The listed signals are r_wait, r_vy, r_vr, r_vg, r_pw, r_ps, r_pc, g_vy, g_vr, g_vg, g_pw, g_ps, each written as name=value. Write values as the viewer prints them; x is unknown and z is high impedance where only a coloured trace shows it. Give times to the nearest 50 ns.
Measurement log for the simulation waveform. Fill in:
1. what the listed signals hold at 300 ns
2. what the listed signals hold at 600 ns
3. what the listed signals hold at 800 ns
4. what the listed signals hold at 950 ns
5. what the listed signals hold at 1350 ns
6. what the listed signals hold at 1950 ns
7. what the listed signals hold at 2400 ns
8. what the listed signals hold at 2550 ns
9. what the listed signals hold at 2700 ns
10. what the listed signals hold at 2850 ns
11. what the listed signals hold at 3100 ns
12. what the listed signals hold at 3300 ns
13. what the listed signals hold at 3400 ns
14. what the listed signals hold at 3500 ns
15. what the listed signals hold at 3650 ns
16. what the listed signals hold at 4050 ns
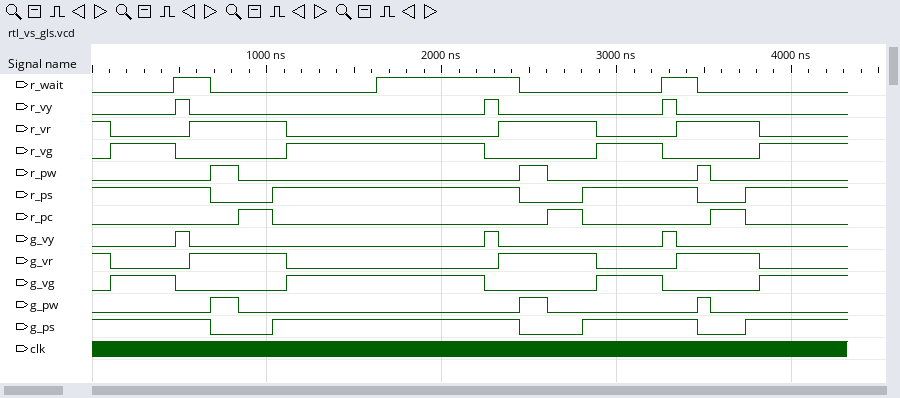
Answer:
r_wait=0, r_vy=0, r_vr=0, r_vg=1, r_pw=0, r_ps=1, r_pc=0, g_vy=0, g_vr=0, g_vg=1, g_pw=0, g_ps=1
r_wait=1, r_vy=0, r_vr=1, r_vg=0, r_pw=0, r_ps=1, r_pc=0, g_vy=0, g_vr=1, g_vg=0, g_pw=0, g_ps=1
r_wait=0, r_vy=0, r_vr=1, r_vg=0, r_pw=1, r_ps=0, r_pc=0, g_vy=0, g_vr=1, g_vg=0, g_pw=1, g_ps=0
r_wait=0, r_vy=0, r_vr=1, r_vg=0, r_pw=0, r_ps=0, r_pc=1, g_vy=0, g_vr=1, g_vg=0, g_pw=0, g_ps=0
r_wait=0, r_vy=0, r_vr=0, r_vg=1, r_pw=0, r_ps=1, r_pc=0, g_vy=0, g_vr=0, g_vg=1, g_pw=0, g_ps=1
r_wait=1, r_vy=0, r_vr=0, r_vg=1, r_pw=0, r_ps=1, r_pc=0, g_vy=0, g_vr=0, g_vg=1, g_pw=0, g_ps=1
r_wait=1, r_vy=0, r_vr=1, r_vg=0, r_pw=0, r_ps=1, r_pc=0, g_vy=0, g_vr=1, g_vg=0, g_pw=0, g_ps=1
r_wait=0, r_vy=0, r_vr=1, r_vg=0, r_pw=1, r_ps=0, r_pc=0, g_vy=0, g_vr=1, g_vg=0, g_pw=1, g_ps=0
r_wait=0, r_vy=0, r_vr=1, r_vg=0, r_pw=0, r_ps=0, r_pc=1, g_vy=0, g_vr=1, g_vg=0, g_pw=0, g_ps=0
r_wait=0, r_vy=0, r_vr=1, r_vg=0, r_pw=0, r_ps=1, r_pc=0, g_vy=0, g_vr=1, g_vg=0, g_pw=0, g_ps=1
r_wait=0, r_vy=0, r_vr=0, r_vg=1, r_pw=0, r_ps=1, r_pc=0, g_vy=0, g_vr=0, g_vg=1, g_pw=0, g_ps=1
r_wait=1, r_vy=1, r_vr=0, r_vg=0, r_pw=0, r_ps=1, r_pc=0, g_vy=1, g_vr=0, g_vg=0, g_pw=0, g_ps=1
r_wait=1, r_vy=0, r_vr=1, r_vg=0, r_pw=0, r_ps=1, r_pc=0, g_vy=0, g_vr=1, g_vg=0, g_pw=0, g_ps=1
r_wait=0, r_vy=0, r_vr=1, r_vg=0, r_pw=1, r_ps=0, r_pc=0, g_vy=0, g_vr=1, g_vg=0, g_pw=1, g_ps=0
r_wait=0, r_vy=0, r_vr=1, r_vg=0, r_pw=0, r_ps=0, r_pc=1, g_vy=0, g_vr=1, g_vg=0, g_pw=0, g_ps=0
r_wait=0, r_vy=0, r_vr=0, r_vg=1, r_pw=0, r_ps=1, r_pc=0, g_vy=0, g_vr=0, g_vg=1, g_pw=0, g_ps=1
